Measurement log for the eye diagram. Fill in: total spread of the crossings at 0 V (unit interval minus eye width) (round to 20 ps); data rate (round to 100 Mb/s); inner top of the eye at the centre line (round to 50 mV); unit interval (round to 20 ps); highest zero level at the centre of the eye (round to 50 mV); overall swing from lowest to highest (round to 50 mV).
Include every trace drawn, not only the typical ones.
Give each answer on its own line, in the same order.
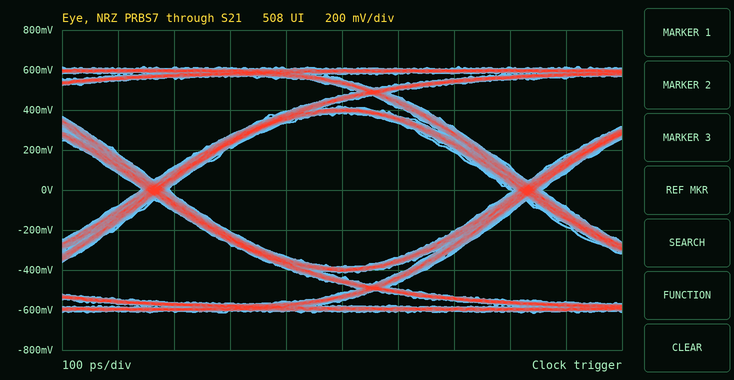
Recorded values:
60 ps
1.5 Gb/s
400 mV
660 ps
-400 mV
1.25 V
